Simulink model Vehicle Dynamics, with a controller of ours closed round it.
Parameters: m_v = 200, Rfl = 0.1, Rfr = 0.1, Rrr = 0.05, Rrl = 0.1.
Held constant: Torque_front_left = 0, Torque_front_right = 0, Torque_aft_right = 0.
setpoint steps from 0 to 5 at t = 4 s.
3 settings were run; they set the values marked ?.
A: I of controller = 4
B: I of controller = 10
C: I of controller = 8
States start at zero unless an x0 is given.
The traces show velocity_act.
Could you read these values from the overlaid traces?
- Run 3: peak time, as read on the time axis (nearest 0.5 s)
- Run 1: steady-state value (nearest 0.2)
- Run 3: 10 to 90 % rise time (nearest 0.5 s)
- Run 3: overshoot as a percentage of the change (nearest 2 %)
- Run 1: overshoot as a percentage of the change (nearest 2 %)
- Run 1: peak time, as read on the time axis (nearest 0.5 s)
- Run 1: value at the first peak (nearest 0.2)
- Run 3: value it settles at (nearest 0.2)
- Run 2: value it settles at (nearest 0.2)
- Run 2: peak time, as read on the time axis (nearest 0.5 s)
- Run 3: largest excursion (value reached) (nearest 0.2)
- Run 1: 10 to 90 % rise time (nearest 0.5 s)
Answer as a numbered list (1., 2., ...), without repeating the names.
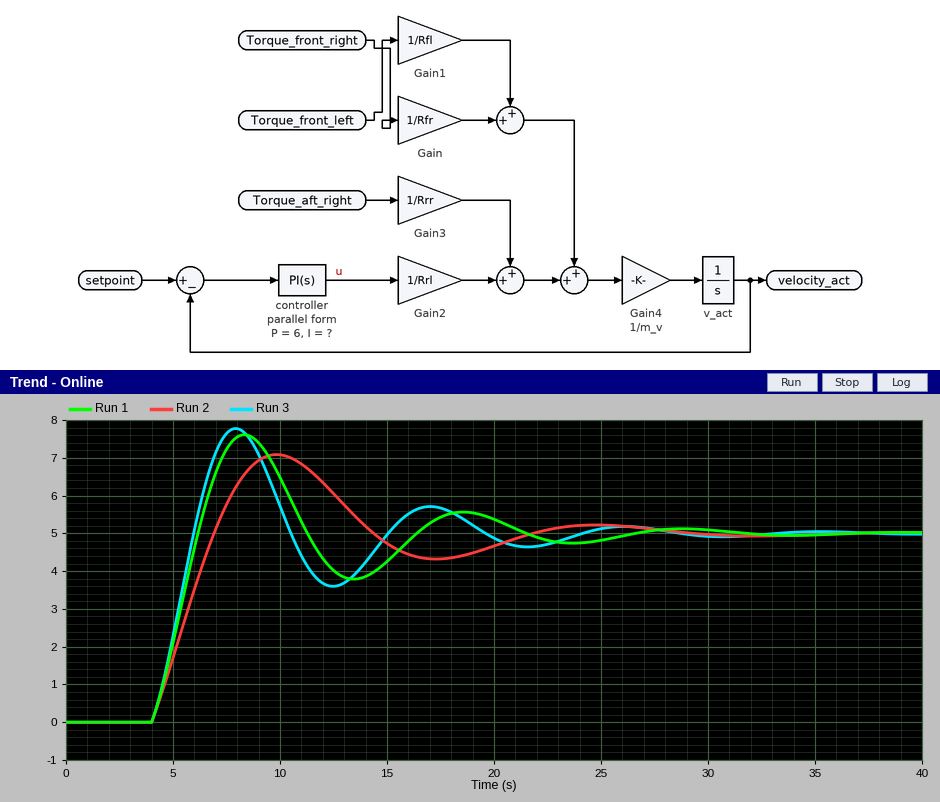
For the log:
1. 8.0 s
2. 5.0
3. 1.5 s
4. 56 %
5. 52 %
6. 8.5 s
7. 7.6
8. 5.0
9. 5.0
10. 10.0 s
11. 7.8
12. 1.5 s
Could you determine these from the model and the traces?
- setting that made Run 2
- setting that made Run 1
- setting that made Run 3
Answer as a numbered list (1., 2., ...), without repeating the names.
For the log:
1. A
2. C
3. B
